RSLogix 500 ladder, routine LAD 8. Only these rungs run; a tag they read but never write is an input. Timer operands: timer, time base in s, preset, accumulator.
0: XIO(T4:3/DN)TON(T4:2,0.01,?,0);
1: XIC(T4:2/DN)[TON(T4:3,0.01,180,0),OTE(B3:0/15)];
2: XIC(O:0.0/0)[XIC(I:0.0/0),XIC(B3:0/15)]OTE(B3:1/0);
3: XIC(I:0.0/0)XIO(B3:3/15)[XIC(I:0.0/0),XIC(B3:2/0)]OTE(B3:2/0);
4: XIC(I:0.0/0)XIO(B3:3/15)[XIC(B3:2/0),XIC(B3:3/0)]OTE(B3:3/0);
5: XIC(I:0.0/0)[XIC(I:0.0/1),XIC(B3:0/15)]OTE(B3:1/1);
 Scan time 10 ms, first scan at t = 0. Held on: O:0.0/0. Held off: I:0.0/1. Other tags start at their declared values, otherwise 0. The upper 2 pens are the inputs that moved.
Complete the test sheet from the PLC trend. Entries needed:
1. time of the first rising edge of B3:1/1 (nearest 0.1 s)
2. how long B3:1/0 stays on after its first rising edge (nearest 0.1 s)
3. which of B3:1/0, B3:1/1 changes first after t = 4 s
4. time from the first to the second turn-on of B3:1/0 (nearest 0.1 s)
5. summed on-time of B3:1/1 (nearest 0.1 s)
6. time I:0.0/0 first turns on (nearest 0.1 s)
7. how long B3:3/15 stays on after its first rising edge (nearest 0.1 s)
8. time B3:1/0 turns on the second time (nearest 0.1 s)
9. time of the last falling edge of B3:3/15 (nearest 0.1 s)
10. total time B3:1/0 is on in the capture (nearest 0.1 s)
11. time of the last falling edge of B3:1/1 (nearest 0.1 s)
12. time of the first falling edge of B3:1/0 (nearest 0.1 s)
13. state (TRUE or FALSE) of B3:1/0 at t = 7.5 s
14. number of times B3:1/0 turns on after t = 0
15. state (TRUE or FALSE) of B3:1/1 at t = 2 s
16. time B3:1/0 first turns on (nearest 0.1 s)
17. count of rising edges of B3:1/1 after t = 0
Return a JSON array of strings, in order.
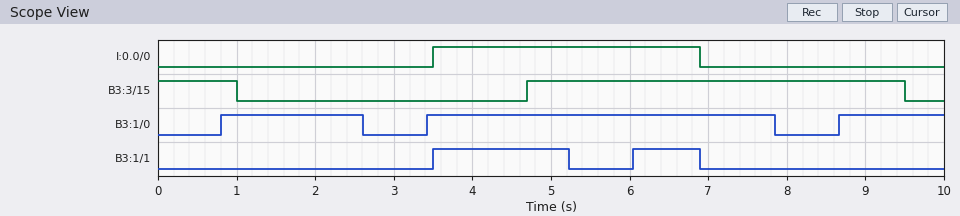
["3.5 s", "1.8 s", "B3:1/1", "2.6 s", "2.6 s", "3.5 s", "4.8 s", "3.4 s", "9.5 s", "7.6 s", "6.9 s", "2.6 s", "TRUE", "3", "FALSE", "0.8 s", "2"]
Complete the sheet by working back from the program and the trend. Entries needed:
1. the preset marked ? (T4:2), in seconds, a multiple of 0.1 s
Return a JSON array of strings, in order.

["0.8 s"]
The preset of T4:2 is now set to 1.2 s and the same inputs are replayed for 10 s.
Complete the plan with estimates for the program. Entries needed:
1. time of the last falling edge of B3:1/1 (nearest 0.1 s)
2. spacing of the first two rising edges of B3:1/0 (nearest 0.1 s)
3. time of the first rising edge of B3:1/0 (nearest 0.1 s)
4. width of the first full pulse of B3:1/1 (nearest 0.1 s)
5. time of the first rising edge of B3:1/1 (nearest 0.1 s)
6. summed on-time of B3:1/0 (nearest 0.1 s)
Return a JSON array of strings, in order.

["6.0 s", "2.3 s", "1.2 s", "1.8 s", "4.2 s", "7.0 s"]
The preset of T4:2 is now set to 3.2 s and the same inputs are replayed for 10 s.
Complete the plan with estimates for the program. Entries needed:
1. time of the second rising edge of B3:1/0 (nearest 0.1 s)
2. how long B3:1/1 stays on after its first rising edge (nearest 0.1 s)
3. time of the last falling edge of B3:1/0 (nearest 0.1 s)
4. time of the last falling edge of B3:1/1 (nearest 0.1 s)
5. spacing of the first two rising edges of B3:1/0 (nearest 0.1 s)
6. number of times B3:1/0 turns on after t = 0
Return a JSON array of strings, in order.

["8.2 s", "1.5 s", "6.9 s", "5.0 s", "5.0 s", "2"]
